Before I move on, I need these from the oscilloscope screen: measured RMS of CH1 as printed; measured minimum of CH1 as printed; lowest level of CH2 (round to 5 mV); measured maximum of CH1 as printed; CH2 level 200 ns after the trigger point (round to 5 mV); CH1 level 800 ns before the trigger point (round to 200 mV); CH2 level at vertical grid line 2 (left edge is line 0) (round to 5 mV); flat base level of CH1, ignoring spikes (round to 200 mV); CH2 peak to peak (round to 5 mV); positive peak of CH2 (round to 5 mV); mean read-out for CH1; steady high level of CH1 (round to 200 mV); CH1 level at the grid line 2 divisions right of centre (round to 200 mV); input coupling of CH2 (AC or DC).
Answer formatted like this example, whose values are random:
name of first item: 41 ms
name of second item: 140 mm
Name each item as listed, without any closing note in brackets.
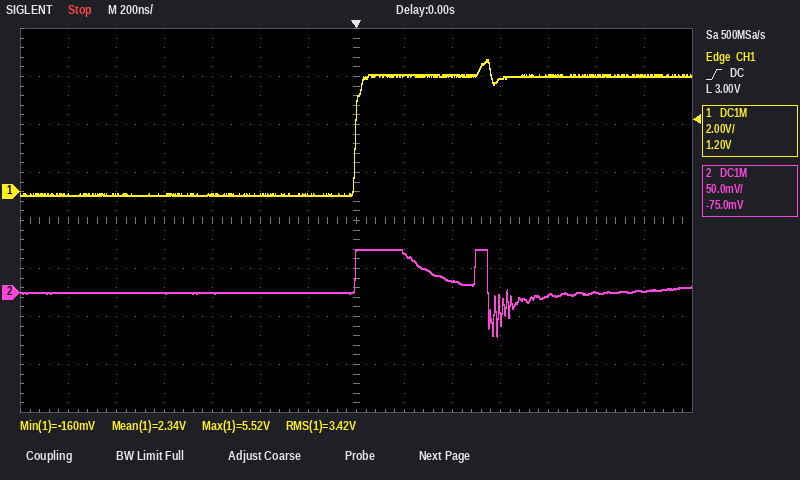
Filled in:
measured RMS of CH1 as printed: 3.42 V
measured minimum of CH1 as printed: -160 mV
lowest level of CH2: -45 mV
measured maximum of CH1 as printed: 5.52 V
CH2 level 200 ns after the trigger point: 40 mV
CH1 level 800 ns before the trigger point: -200 mV
CH2 level at vertical grid line 2 (left edge is line 0): 0 mV
flat base level of CH1, ignoring spikes: -200 mV
CH2 peak to peak: 90 mV
positive peak of CH2: 45 mV
mean read-out for CH1: 2.34 V
steady high level of CH1: 4.8 V
CH1 level at the grid line 2 divisions right of centre: 4.8 V
input coupling of CH2: DC
